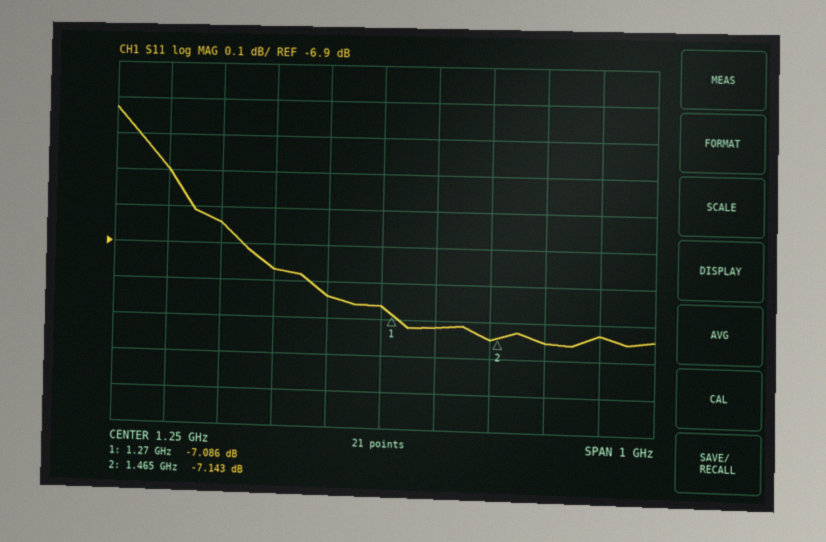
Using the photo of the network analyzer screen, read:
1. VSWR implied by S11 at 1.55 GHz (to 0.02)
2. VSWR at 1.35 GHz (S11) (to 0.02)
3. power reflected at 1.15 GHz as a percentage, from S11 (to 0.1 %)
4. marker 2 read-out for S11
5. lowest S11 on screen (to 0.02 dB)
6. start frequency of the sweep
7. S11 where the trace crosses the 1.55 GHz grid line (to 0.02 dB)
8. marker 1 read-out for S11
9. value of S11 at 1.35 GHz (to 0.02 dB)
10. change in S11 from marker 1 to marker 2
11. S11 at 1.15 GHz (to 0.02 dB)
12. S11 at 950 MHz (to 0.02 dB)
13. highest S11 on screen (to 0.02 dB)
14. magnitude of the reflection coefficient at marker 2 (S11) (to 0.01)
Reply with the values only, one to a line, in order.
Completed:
2.56
2.58
19.8 %
-7.143 dB
-7.16 dB
750 MHz
-7.16 dB
-7.086 dB
-7.12 dB
-0.057 dB
-7.04 dB
-6.84 dB
-6.52 dB
0.44
